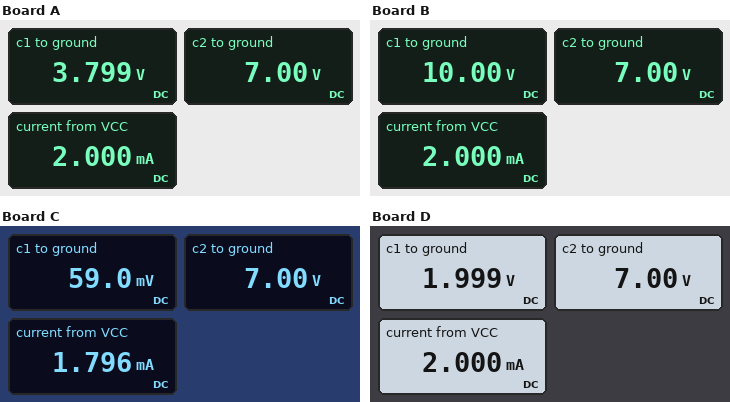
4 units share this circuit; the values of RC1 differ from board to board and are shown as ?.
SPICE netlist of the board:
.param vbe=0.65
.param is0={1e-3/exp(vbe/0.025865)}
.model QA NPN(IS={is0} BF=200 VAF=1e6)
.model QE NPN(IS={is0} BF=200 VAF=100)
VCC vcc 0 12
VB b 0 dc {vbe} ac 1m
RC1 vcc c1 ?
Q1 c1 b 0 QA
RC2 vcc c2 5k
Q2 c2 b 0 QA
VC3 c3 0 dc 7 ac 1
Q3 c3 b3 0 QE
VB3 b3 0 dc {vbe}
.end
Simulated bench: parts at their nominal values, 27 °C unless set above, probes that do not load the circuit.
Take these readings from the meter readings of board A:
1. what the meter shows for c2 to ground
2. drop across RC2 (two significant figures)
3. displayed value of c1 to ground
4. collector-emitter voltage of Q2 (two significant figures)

7.00 V
5.0 V
3.799 V
7.0 V
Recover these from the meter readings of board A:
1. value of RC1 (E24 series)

8.2 kΩ
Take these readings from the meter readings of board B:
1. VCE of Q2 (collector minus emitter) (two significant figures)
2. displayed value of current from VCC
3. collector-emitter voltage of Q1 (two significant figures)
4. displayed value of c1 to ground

7.0 V
2.000 mA
10 V
10.00 V
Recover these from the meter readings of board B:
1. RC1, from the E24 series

2 kΩ
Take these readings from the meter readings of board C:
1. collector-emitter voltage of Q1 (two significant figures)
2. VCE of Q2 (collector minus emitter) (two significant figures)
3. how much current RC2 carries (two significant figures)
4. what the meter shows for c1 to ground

59 mV
7.0 V
1.0 mA
59.0 mV
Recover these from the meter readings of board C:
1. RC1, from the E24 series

15 kΩ
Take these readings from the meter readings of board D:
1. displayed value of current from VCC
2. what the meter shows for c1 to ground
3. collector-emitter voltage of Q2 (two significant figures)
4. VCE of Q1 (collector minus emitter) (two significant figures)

2.000 mA
1.999 V
7.0 V
2.0 V
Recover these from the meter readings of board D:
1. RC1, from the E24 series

10 kΩ
